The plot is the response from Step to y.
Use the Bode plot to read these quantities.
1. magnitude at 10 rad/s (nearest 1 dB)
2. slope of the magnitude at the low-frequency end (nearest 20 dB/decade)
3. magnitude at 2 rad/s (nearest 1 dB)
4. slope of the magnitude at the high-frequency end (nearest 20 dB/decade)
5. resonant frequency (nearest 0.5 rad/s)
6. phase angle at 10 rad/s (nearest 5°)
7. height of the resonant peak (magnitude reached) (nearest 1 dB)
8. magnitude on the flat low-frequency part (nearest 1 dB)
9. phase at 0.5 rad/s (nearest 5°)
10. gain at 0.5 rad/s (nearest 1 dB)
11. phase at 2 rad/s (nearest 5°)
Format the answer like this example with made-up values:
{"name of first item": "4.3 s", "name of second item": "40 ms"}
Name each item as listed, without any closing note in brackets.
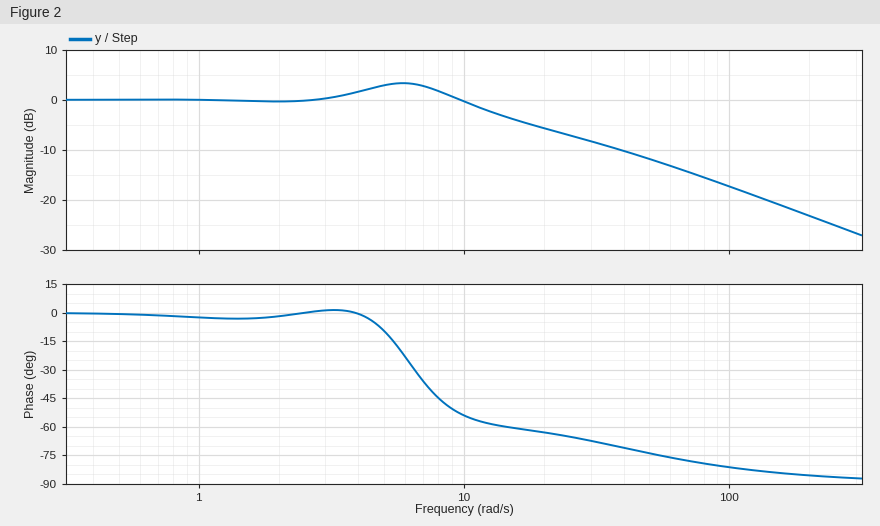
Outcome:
{"magnitude at 10 rad/s": "0 dB", "slope of the magnitude at the low-frequency end": "0 dB/decade", "magnitude at 2 rad/s": "0 dB", "slope of the magnitude at the high-frequency end": "-20 dB/decade", "resonant frequency": "6.0 rad/s", "phase angle at 10 rad/s": "-55°", "height of the resonant peak (magnitude reached)": "3 dB", "magnitude on the flat low-frequency part": "0 dB", "phase at 0.5 rad/s": "0°", "gain at 0.5 rad/s": "0 dB", "phase at 2 rad/s": "0°"}
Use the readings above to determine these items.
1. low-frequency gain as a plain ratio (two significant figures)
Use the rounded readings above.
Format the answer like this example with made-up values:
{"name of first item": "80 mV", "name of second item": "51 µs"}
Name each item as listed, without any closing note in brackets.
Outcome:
{"low-frequency gain as a plain ratio": "1.0"}
